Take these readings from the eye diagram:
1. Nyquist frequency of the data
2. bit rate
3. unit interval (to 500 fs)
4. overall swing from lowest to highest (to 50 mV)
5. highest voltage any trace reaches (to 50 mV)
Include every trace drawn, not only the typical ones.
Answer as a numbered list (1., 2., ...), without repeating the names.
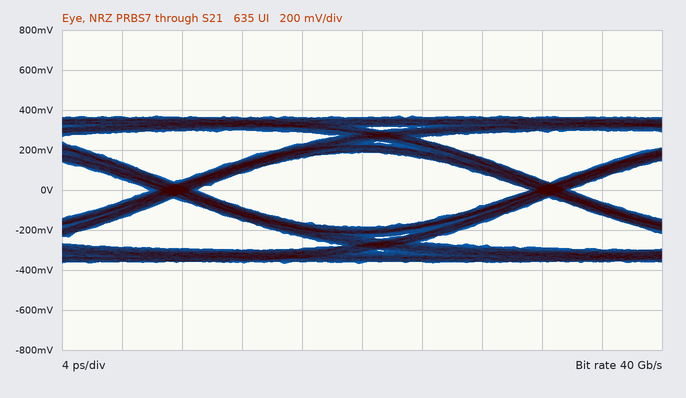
1. 20 GHz
2. 40 Gb/s
3. 25.0 ps
4. 750 mV
5. 350 mV
